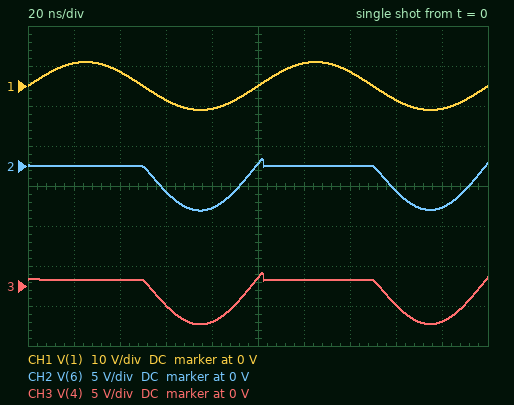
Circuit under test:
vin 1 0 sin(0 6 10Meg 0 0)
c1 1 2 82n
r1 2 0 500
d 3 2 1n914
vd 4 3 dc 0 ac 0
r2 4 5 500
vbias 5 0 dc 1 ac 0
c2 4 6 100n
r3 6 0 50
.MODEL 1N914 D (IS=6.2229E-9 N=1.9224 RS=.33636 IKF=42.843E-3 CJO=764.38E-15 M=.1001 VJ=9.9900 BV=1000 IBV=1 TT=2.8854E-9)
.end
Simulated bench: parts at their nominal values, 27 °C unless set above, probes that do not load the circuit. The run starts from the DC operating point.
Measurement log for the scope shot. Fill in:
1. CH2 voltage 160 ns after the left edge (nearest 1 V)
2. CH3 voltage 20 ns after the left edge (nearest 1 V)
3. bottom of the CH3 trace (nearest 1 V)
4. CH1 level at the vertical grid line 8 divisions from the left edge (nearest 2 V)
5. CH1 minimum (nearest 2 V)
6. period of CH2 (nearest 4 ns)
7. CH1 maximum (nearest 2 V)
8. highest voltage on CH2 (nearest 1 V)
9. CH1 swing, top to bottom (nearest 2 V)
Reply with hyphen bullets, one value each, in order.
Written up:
- -3 V
- 1 V
- -5 V
- -4 V
- -6 V
- 100 ns
- 6 V
- 1 V
- 12 V
